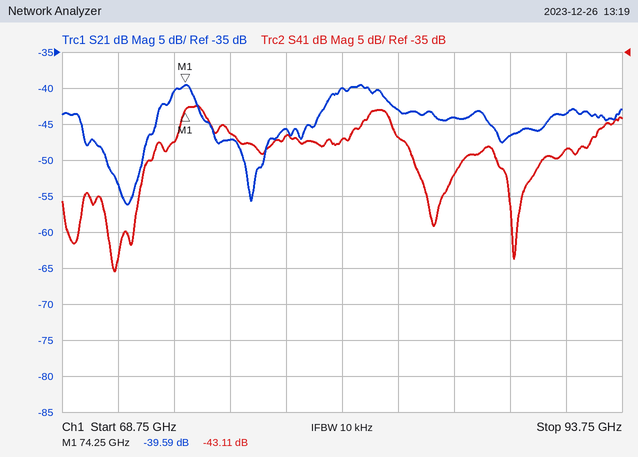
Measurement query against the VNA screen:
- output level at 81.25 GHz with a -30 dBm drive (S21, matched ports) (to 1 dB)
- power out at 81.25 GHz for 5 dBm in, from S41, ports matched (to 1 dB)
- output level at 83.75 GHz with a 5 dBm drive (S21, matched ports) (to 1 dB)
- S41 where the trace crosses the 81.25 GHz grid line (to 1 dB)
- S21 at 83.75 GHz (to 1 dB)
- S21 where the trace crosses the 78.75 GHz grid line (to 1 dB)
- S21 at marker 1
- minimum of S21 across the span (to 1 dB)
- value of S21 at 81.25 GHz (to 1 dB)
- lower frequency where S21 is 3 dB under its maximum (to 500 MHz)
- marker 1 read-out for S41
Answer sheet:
-70 dBm
-42 dBm
-38 dBm
-47 dB
-43 dB
-46 dB
-39.59 dB
-56 dB
-40 dB
73.0 GHz
-43.11 dB
